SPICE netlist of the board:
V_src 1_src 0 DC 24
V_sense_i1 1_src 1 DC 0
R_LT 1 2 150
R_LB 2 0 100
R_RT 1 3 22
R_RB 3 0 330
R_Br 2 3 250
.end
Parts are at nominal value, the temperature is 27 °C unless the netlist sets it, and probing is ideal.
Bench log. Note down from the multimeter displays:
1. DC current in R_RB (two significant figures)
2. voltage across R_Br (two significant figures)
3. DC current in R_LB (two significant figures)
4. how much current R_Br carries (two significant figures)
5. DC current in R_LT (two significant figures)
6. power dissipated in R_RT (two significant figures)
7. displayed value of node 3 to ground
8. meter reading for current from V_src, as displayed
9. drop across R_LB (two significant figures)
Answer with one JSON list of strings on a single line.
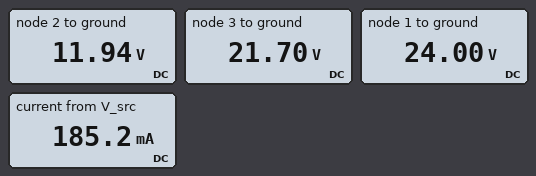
["66 mA", "9.8 V", "120 mA", "39 mA", "80 mA", "240 mW", "21.70 V", "185.2 mA", "12 V"]
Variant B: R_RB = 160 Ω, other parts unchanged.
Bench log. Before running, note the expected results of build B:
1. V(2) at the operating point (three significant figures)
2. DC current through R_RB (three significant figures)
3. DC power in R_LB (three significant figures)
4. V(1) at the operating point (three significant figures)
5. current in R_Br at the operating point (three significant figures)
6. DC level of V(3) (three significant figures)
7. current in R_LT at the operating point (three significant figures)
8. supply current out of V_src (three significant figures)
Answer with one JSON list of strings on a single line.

["11.7 V", "128 mA", "1.37 W", "24.0 V", "34.9 mA", "20.4 V", "82.0 mA", "245 mA"]
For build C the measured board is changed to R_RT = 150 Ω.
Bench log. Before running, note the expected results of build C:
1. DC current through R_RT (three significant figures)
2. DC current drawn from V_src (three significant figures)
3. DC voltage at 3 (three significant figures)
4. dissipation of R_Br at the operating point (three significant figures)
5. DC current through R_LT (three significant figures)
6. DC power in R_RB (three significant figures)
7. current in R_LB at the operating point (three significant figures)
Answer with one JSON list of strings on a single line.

["61.5 mA", "151 mA", "14.8 V", "69.7 mW", "89.3 mA", "662 mW", "106 mA"]
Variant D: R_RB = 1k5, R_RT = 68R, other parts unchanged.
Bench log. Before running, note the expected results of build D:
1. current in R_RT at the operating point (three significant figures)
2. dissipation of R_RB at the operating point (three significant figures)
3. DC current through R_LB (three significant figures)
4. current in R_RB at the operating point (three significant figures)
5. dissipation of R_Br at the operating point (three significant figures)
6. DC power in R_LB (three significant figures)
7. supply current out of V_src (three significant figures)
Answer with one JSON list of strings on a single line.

["49.4 mA", "284 mW", "117 mA", "13.8 mA", "317 mW", "1.38 W", "131 mA"]
